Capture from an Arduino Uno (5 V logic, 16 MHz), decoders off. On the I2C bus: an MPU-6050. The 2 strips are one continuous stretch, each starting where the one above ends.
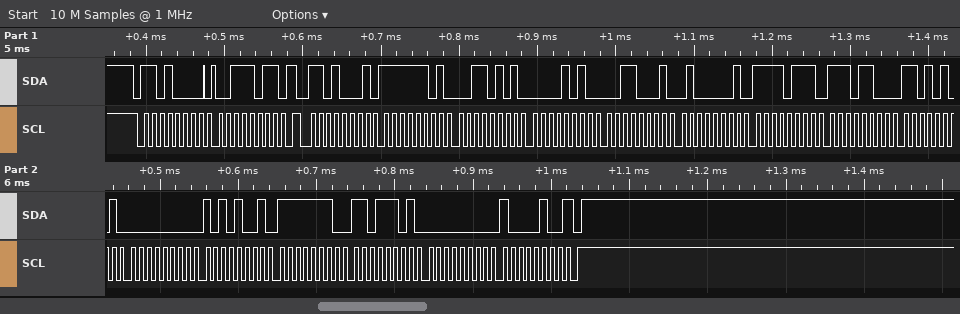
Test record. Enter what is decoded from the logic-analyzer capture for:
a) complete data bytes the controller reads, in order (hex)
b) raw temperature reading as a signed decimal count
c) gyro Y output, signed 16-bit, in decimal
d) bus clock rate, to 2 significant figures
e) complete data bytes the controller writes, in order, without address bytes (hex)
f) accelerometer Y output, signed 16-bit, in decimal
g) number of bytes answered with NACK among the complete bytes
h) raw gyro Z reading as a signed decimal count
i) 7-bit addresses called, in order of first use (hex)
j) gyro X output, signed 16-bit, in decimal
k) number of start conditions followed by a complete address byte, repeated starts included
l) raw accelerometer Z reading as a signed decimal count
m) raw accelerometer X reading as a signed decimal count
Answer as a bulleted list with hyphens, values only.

- FD 35 0A 31 41 F7 EC D5 00 A9 FE DD 00 84
- -4907
- -291
- 100 kHz
- 3B
- 2609
- 1
- 132
- 0x68
- 169
- 2
- 16887
- -715
